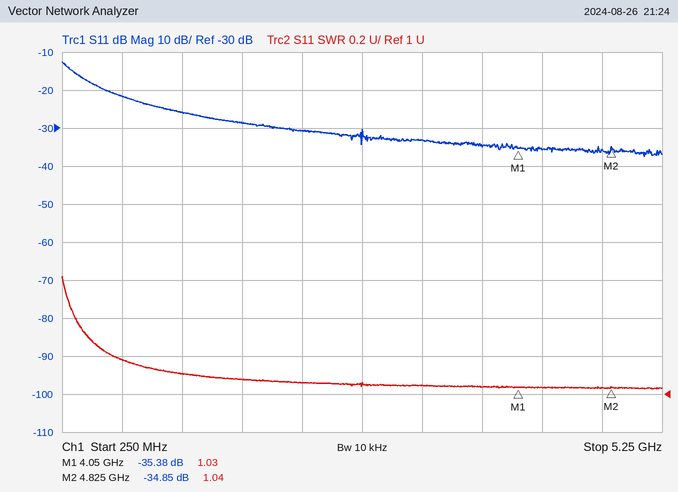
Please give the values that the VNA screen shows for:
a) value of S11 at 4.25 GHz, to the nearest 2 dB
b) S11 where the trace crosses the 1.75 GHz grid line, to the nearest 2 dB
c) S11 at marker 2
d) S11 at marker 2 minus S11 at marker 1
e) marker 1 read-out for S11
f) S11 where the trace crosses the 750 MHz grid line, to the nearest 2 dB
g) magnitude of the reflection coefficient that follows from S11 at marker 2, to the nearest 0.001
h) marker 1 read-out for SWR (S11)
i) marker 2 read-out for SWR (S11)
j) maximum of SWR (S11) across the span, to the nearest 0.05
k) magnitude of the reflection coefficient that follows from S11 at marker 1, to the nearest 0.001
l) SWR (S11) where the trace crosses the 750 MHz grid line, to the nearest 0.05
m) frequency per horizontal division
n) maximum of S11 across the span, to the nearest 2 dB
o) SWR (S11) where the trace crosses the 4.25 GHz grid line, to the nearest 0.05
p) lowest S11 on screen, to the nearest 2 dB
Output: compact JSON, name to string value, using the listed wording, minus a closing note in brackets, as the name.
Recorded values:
{"value of S11 at 4.25 GHz, to the nearest 2 dB": "-36 dB", "S11 where the trace crosses the 1.75 GHz grid line, to the nearest 2 dB": "-28 dB", "S11 at marker 2": "-34.85 dB", "S11 at marker 2 minus S11 at marker 1": "0.53 dB", "marker 1 read-out for S11": "-35.38 dB", "S11 where the trace crosses the 750 MHz grid line, to the nearest 2 dB": "-22 dB", "magnitude of the reflection coefficient that follows from S11 at marker 2, to the nearest 0.001": "0.018", "marker 1 read-out for SWR": "1.03", "marker 2 read-out for SWR": "1.04", "maximum of SWR (S11) across the span, to the nearest 0.05": "1.60", "magnitude of the reflection coefficient that follows from S11 at marker 1, to the nearest 0.001": "0.017", "SWR (S11) where the trace crosses the 750 MHz grid line, to the nearest 0.05": "1.20", "frequency per horizontal division": "500 MHz", "maximum of S11 across the span, to the nearest 2 dB": "-12 dB", "SWR (S11) where the trace crosses the 4.25 GHz grid line, to the nearest 0.05": "1.05", "lowest S11 on screen, to the nearest 2 dB": "-38 dB"}
